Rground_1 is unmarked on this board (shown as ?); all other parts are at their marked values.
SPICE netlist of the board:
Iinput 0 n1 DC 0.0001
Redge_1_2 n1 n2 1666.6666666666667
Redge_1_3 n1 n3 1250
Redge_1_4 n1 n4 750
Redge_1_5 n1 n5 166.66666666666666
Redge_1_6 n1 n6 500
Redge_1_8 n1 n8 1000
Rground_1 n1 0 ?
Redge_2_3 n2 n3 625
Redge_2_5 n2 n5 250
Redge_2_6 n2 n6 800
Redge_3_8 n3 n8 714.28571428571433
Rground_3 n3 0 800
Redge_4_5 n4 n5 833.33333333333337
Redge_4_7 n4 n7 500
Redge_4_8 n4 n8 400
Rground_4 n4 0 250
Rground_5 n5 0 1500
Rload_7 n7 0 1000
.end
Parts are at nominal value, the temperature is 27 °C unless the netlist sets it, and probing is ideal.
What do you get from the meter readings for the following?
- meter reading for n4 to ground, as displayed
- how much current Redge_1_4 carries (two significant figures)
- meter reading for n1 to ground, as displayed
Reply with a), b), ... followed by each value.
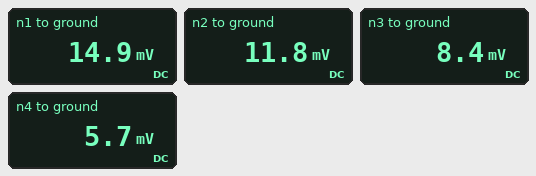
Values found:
a) 5.7 mV
b) 12 µA
c) 14.9 mV
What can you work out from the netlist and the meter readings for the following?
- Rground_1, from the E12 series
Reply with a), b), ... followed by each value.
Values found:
a) 270 Ω
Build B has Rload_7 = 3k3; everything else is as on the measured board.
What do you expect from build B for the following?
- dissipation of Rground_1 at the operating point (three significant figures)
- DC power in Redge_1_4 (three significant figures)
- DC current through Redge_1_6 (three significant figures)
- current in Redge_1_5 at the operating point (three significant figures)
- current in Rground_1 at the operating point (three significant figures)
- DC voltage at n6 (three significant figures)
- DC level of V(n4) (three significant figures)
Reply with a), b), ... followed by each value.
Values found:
a) 832 nW
b) 107 nW
c) 2.37 µA
d) 16.7 µA
e) 55.5 µA
f) 13.8 mV
g) 6.03 mV
